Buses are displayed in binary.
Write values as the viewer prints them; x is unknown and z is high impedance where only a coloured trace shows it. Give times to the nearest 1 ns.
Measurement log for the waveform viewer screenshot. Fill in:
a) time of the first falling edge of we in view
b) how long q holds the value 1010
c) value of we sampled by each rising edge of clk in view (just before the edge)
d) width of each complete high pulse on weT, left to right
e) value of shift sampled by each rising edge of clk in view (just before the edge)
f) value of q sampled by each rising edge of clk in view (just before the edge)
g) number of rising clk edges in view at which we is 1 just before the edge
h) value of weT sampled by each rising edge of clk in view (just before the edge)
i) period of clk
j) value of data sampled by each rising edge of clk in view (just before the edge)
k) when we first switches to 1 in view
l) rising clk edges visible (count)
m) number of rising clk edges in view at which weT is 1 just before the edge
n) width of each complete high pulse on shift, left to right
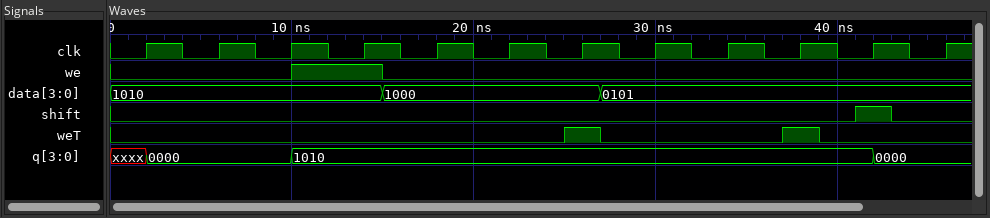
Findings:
15 ns
32 ns
0 0 0 1 0 0 0 0 0 0 0 0
2 ns, 2 ns
0 0 0 0 0 0 0 0 0 0 1 0
xxxx, 0000, 0000, 1010, 1010, 1010, 1010, 1010, 1010, 1010, 1010, 0000
1
0 0 0 0 0 0 1 0 0 1 0 0
4 ns
1010, 1010, 1010, 1010, 1000, 1000, 1000, 0101, 0101, 0101, 0101, 0101
10 ns
12
2
2 ns
